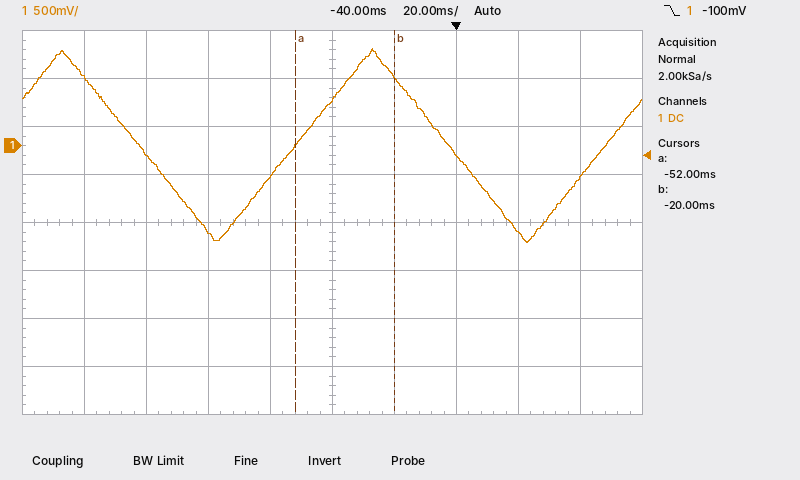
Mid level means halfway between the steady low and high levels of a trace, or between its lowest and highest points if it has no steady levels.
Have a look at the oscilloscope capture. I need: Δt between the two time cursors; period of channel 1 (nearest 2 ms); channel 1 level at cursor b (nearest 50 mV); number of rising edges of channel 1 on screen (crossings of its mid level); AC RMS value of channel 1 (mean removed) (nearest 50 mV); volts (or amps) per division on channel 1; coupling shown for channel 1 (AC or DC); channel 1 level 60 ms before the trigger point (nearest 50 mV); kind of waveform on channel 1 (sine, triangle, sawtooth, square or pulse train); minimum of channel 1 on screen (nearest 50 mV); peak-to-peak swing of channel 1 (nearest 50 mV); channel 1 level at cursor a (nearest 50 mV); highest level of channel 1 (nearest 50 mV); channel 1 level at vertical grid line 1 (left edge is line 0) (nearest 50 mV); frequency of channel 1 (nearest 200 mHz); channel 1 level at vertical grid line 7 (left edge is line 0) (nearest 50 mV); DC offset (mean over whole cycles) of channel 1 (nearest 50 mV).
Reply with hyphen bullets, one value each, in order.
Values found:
- 32 ms
- 100 ms
- 700 mV
- 2
- 600 mV
- 500 mV
- DC
- -300 mV
- triangle
- -1.00 V
- 2.00 V
- 0 mV
- 1.00 V
- 700 mV
- 10.0 Hz
- -100 mV
- 0 mV
